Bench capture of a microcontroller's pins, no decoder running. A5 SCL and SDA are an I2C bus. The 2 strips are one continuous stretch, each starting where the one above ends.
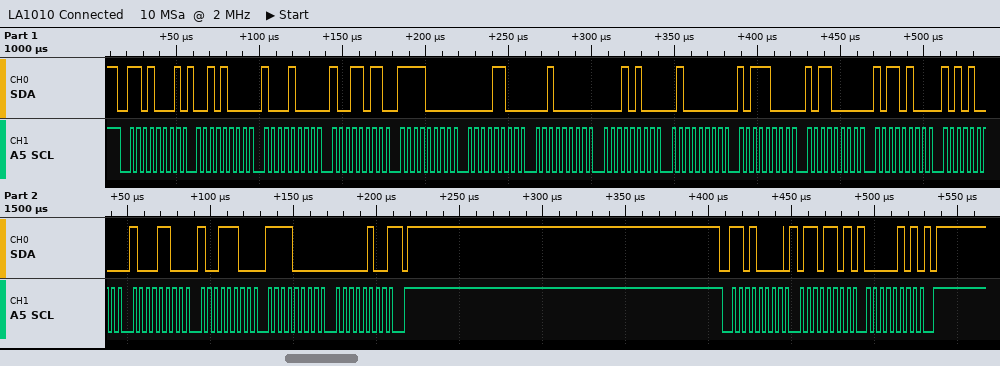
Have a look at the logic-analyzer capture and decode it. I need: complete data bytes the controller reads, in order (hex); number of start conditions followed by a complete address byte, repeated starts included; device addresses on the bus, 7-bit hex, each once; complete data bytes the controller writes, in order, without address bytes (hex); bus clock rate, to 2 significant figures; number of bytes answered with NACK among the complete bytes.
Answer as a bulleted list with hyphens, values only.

- 28 88 9B F0 0C 20 14 40 B8 B0 B4 A8 8C 9C F0 04
- 2
- 0x68
- 6D 05
- 250 kHz
- 1
